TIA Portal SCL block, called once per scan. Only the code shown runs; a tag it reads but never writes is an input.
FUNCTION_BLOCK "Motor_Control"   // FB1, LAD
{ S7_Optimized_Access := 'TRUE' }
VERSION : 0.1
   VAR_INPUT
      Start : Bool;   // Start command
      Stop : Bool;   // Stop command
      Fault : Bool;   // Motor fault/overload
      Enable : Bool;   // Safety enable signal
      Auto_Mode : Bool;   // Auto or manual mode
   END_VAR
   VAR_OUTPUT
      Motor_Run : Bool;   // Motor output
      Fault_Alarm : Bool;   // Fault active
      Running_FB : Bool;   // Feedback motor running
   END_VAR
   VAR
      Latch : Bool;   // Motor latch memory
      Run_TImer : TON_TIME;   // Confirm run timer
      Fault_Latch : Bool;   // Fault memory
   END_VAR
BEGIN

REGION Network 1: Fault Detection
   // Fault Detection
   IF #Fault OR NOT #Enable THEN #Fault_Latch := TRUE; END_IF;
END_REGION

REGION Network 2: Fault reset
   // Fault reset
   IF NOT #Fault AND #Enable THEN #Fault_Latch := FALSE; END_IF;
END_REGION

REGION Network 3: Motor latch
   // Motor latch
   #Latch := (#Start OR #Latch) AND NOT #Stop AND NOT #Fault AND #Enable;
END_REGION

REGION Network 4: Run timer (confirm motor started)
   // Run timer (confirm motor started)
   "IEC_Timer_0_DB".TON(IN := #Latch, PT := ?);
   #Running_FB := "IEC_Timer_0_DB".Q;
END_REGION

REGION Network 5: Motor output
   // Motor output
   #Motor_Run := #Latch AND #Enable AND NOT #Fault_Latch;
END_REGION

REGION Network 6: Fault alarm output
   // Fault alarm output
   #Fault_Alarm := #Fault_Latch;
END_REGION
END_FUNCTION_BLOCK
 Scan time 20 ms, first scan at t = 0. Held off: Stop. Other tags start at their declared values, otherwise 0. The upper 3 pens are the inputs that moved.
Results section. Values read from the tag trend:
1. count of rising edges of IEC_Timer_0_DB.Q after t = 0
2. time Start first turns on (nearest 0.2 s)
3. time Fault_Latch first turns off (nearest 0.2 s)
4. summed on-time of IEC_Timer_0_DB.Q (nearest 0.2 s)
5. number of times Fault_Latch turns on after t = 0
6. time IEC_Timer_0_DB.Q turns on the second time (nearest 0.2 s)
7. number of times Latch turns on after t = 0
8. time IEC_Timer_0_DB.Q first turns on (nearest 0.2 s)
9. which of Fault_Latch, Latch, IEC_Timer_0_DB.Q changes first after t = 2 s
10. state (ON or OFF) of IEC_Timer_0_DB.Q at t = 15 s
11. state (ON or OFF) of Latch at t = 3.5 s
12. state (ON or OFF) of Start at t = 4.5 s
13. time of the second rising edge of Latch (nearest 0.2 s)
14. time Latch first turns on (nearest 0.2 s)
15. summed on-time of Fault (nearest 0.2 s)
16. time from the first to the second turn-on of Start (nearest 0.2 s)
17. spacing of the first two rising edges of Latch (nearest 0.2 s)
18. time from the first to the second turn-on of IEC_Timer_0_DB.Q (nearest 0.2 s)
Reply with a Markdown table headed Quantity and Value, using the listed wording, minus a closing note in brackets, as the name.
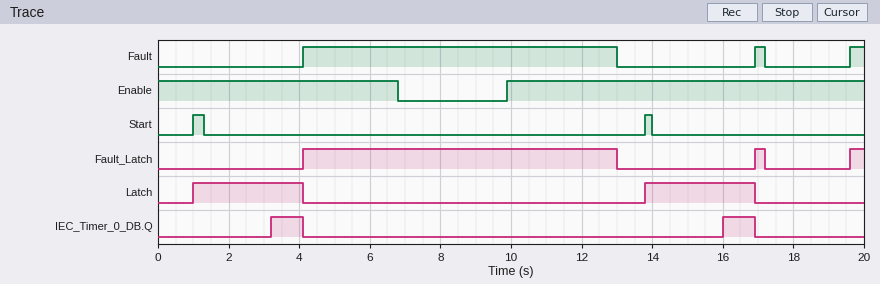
| Quantity | Value |
|---|---|
| count of rising edges of IEC_Timer_0_DB.Q after t = 0 | 2 |
| time Start first turns on | 1.0 s |
| time Fault_Latch first turns off | 13.0 s |
| summed on-time of IEC_Timer_0_DB.Q | 1.8 s |
| number of times Fault_Latch turns on after t = 0 | 3 |
| time IEC_Timer_0_DB.Q turns on the second time | 16.0 s |
| number of times Latch turns on after t = 0 | 2 |
| time IEC_Timer_0_DB.Q first turns on | 3.2 s |
| which of Fault_Latch, Latch, IEC_Timer_0_DB.Q changes first after t = 2 s | IEC_Timer_0_DB.Q |
| state (ON or OFF) of IEC_Timer_0_DB.Q at t = 15 s | OFF |
| state (ON or OFF) of Latch at t = 3.5 s | ON |
| state (ON or OFF) of Start at t = 4.5 s | OFF |
| time of the second rising edge of Latch | 13.8 s |
| time Latch first turns on | 1.0 s |
| summed on-time of Fault | 9.6 s |
| time from the first to the second turn-on of Start | 12.8 s |
| spacing of the first two rising edges of Latch | 12.8 s |
| time from the first to the second turn-on of IEC_Timer_0_DB.Q | 12.8 s |
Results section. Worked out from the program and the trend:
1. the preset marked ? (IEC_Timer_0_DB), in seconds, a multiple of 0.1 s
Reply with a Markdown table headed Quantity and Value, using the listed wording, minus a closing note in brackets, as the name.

| Quantity | Value |
|---|---|
| the preset marked ? (IEC_Timer_0_DB), in seconds, a multiple of 0.1 s | 2.2 s |
